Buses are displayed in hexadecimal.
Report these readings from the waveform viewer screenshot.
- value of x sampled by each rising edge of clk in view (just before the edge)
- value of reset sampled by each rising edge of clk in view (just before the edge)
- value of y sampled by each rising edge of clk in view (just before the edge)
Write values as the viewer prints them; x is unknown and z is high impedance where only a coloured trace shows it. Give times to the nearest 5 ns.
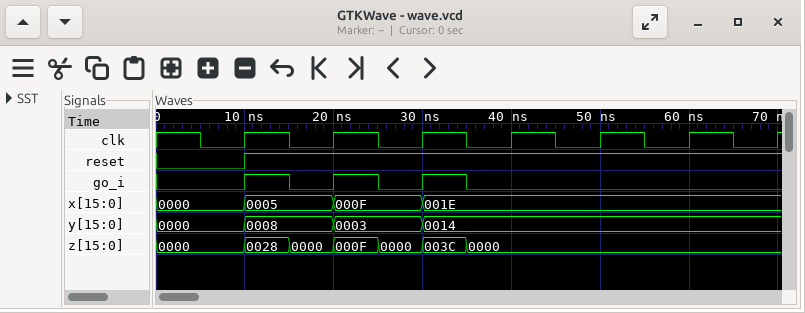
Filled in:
0000, 0005, 000F, 001E, 001E, 001E, 001E
0 1 1 1 1 1 1
0000, 0008, 0003, 0014, 0014, 0014, 0014
